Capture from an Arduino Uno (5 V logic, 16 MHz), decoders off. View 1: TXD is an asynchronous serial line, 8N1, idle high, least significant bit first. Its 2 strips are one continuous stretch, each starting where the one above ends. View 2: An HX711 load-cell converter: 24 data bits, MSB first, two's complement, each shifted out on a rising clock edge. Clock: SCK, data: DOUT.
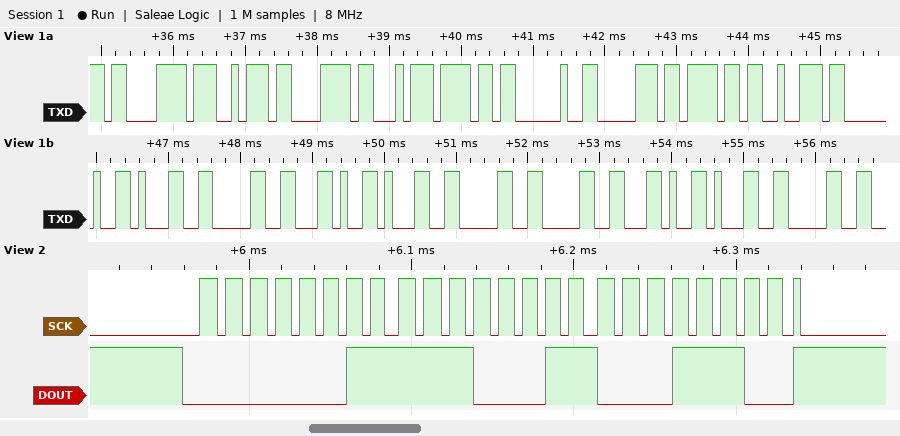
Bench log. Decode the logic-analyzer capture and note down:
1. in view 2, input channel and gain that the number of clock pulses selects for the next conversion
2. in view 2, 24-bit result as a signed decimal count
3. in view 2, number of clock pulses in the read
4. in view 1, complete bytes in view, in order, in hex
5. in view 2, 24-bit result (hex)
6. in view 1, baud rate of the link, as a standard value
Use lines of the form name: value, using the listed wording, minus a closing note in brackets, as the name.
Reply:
in view 2, input channel and gain that the number of clock pulses selects for the next conversion: channel A, gain 128
in view 2, 24-bit result as a signed decimal count: 254748
in view 2, number of clock pulses in the read: 25
in view 1, complete bytes in view, in order, in hex: C3 A7 C3 A3 6F 20 70 6F 72 20 31 30 2C 31 30 30 2C 31 30
in view 2, 24-bit result: 0x03E31C
in view 1, baud rate of the link, as a standard value: 9600 baud
